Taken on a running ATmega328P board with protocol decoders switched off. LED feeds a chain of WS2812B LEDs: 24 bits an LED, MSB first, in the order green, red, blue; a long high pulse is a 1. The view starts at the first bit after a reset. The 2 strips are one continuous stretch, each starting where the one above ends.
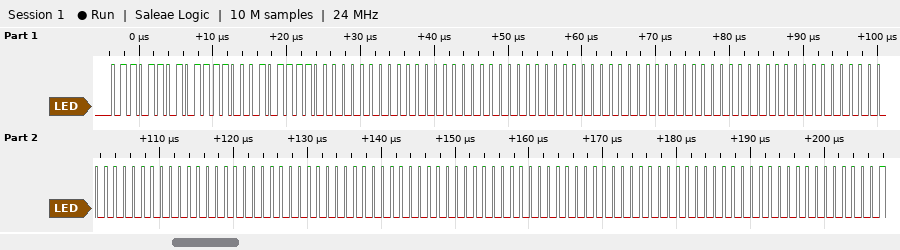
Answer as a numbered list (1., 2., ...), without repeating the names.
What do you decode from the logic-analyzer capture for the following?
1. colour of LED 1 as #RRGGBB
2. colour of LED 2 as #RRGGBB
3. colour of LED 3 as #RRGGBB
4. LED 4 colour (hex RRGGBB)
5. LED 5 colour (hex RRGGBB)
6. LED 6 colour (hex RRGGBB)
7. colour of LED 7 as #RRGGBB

1. #786DBC
2. #000000
3. #000000
4. #000000
5. #000000
6. #000000
7. #000000
